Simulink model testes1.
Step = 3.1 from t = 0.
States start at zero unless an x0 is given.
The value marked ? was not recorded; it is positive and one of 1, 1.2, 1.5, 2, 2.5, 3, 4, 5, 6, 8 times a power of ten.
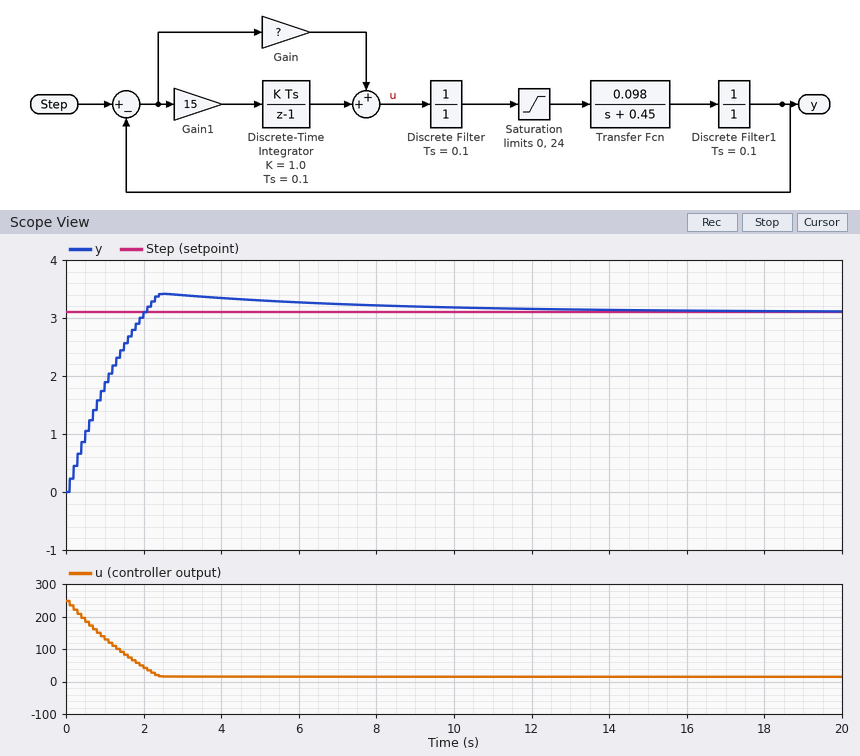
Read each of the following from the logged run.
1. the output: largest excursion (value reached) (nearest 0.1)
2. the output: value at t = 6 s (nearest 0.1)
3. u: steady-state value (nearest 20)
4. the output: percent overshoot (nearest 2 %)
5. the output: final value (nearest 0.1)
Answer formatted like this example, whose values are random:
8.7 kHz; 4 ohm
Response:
3.4; 3.3; 20; 10 %; 3.1
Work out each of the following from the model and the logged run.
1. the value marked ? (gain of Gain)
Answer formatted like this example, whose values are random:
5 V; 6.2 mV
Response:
80
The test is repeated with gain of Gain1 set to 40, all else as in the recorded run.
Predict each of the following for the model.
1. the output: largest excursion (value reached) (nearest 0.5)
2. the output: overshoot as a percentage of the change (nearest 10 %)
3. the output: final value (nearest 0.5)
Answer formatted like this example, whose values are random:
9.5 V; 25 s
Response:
4.0; 30 %; 3.0
